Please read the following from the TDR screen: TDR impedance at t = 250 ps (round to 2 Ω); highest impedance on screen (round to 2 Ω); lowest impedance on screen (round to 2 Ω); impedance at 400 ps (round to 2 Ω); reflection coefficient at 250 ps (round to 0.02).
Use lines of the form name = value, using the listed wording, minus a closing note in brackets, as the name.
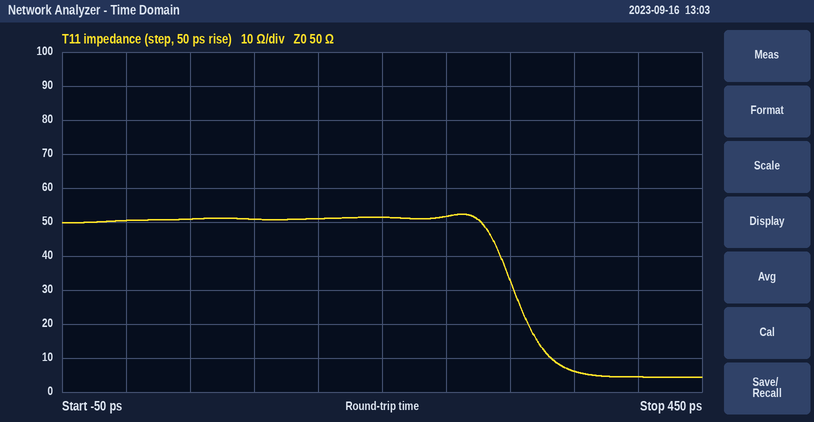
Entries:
TDR impedance at t = 250 ps = 52 Ω
highest impedance on screen = 52 Ω
lowest impedance on screen = 4 Ω
impedance at 400 ps = 4 Ω
reflection coefficient at 250 ps = +0.02
